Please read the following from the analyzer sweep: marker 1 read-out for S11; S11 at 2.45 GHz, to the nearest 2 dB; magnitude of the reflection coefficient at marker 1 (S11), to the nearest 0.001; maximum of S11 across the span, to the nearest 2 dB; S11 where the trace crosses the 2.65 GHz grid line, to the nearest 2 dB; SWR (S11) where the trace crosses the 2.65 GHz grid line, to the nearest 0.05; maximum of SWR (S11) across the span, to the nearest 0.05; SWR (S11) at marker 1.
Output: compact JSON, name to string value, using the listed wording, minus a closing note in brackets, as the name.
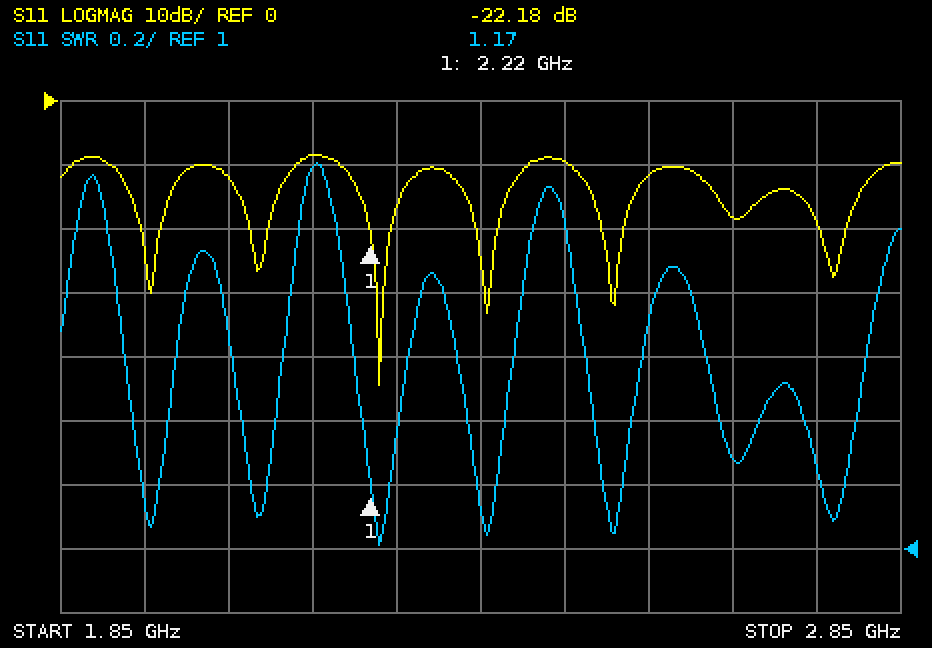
{"marker 1 read-out for S11": "-22.18 dB", "S11 at 2.45 GHz, to the nearest 2 dB": "-10 dB", "magnitude of the reflection coefficient at marker 1 (S11), to the nearest 0.001": "0.078", "maximum of S11 across the span, to the nearest 2 dB": "-8 dB", "S11 where the trace crosses the 2.65 GHz grid line, to the nearest 2 dB": "-18 dB", "SWR (S11) where the trace crosses the 2.65 GHz grid line, to the nearest 0.05": "1.30", "maximum of SWR (S11) across the span, to the nearest 0.05": "2.20", "SWR (S11) at marker 1": "1.17"}
